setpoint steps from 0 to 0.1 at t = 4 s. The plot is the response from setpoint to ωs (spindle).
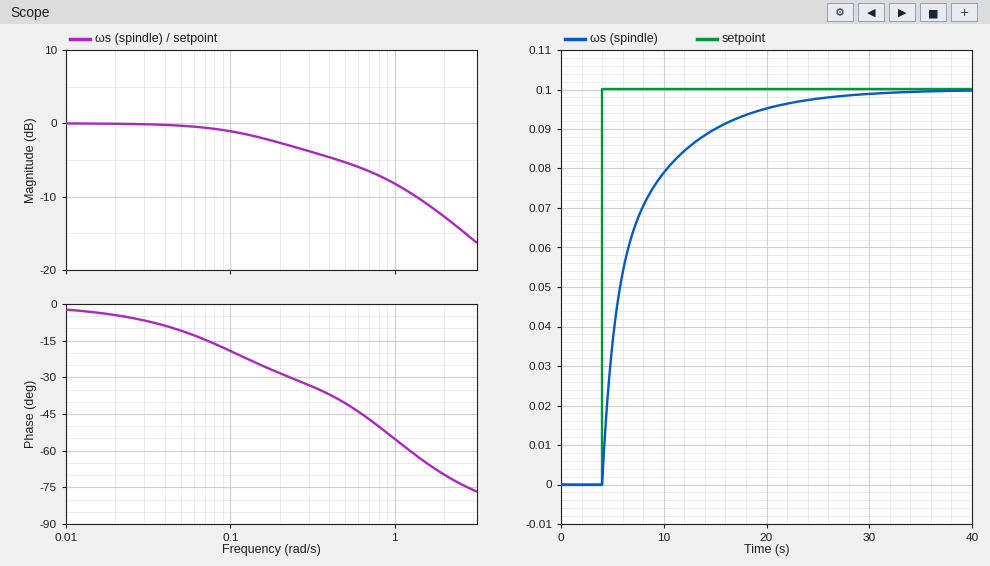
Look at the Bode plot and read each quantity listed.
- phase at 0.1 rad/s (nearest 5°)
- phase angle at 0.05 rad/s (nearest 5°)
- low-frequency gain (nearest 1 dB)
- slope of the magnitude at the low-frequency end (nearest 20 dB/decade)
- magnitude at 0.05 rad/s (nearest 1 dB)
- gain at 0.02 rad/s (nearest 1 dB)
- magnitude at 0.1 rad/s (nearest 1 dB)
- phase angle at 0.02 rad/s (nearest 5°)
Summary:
-20°
-10°
0 dB
0 dB/decade
0 dB
0 dB
-1 dB
-5°
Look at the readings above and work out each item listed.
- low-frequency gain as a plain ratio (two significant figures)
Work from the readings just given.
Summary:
1.0
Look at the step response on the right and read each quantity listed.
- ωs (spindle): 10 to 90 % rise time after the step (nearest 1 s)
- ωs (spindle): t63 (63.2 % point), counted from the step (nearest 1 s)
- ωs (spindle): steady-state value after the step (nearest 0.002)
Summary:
11 s
3 s
0.100
